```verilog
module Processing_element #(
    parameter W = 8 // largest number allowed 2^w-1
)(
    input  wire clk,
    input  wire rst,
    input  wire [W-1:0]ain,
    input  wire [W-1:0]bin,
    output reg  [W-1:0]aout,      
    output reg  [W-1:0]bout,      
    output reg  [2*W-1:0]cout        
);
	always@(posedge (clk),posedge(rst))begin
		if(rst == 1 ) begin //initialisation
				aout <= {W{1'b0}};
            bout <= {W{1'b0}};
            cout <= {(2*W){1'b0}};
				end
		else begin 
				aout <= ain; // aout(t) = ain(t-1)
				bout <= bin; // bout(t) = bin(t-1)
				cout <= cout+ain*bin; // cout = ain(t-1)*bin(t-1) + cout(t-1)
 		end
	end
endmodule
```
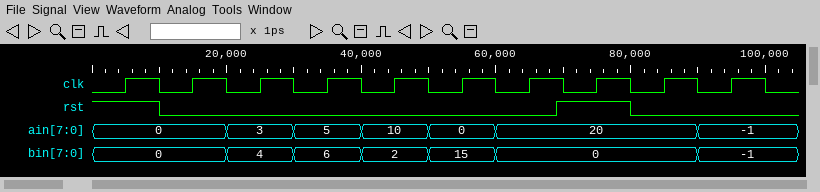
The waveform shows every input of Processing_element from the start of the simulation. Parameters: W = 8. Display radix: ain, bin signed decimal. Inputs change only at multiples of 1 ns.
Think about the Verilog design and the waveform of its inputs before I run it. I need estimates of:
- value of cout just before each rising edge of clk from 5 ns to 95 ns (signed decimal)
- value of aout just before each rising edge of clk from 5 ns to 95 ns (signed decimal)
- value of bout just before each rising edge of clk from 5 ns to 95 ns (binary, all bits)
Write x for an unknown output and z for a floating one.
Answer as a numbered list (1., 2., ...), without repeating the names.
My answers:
1. 0, 0, 0, 12, 42, 62, 62, 0, 0, 0
2. 0, 0, 0, 3, 5, 10, 0, 0, 0, 20
3. 00000000, 00000000, 00000000, 00000100, 00000110, 00000010, 00001111, 00000000, 00000000, 00000000
